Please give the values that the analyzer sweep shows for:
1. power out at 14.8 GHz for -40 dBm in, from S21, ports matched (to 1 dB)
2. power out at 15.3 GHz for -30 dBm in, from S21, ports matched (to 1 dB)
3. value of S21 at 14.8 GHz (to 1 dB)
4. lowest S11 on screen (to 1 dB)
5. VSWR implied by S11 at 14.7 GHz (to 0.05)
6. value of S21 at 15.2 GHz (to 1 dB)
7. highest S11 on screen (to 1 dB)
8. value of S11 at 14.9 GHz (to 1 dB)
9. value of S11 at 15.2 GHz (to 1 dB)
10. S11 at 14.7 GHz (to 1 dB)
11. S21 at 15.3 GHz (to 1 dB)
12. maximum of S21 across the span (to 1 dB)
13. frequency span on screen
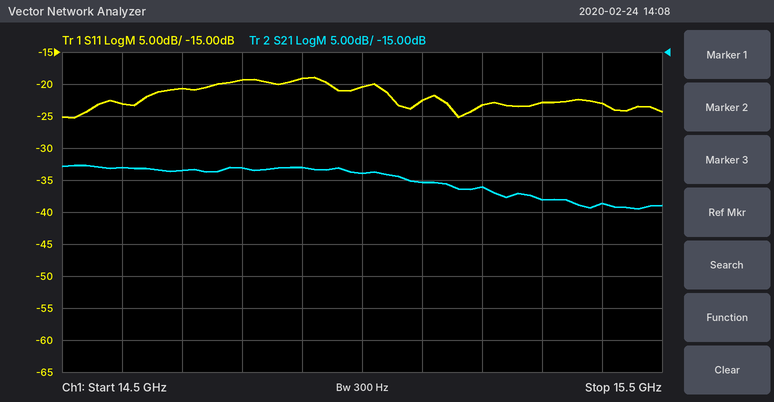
-73 dBm
-68 dBm
-33 dB
-25 dB
1.20
-36 dB
-19 dB
-19 dB
-23 dB
-21 dB
-38 dB
-33 dB
1 GHz
